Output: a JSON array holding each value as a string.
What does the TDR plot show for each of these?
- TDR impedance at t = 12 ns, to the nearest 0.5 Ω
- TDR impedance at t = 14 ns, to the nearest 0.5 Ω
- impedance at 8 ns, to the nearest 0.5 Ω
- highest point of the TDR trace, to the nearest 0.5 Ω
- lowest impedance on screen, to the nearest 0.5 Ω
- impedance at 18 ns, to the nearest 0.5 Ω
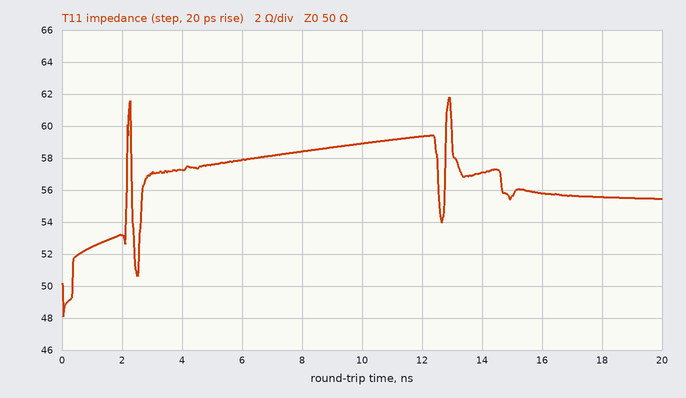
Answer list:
["59.5 Ω", "57.0 Ω", "58.5 Ω", "62.0 Ω", "48.0 Ω", "55.5 Ω"]
